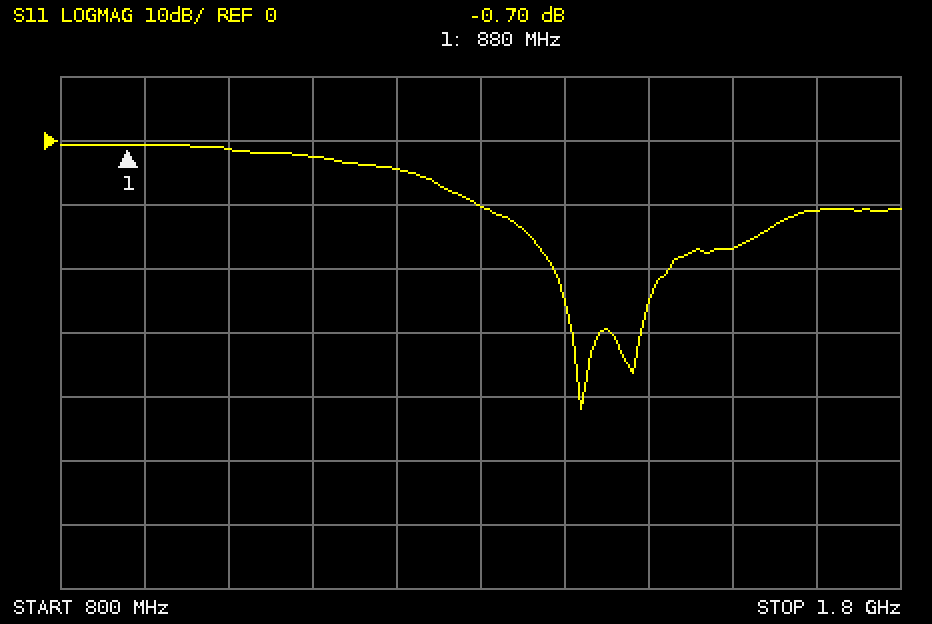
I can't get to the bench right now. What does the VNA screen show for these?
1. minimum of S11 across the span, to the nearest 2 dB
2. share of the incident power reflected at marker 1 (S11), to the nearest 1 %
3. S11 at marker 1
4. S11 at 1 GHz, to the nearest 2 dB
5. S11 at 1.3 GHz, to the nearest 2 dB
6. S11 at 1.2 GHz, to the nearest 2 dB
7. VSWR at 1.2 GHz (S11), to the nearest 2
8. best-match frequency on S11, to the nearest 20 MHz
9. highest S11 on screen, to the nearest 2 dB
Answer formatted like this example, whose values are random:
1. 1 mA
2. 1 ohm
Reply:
1. -42 dB
2. 85 %
3. -0.70 dB
4. -2 dB
5. -10 dB
6. -4 dB
7. 4
8. 1.42 GHz
9. 0 dB
